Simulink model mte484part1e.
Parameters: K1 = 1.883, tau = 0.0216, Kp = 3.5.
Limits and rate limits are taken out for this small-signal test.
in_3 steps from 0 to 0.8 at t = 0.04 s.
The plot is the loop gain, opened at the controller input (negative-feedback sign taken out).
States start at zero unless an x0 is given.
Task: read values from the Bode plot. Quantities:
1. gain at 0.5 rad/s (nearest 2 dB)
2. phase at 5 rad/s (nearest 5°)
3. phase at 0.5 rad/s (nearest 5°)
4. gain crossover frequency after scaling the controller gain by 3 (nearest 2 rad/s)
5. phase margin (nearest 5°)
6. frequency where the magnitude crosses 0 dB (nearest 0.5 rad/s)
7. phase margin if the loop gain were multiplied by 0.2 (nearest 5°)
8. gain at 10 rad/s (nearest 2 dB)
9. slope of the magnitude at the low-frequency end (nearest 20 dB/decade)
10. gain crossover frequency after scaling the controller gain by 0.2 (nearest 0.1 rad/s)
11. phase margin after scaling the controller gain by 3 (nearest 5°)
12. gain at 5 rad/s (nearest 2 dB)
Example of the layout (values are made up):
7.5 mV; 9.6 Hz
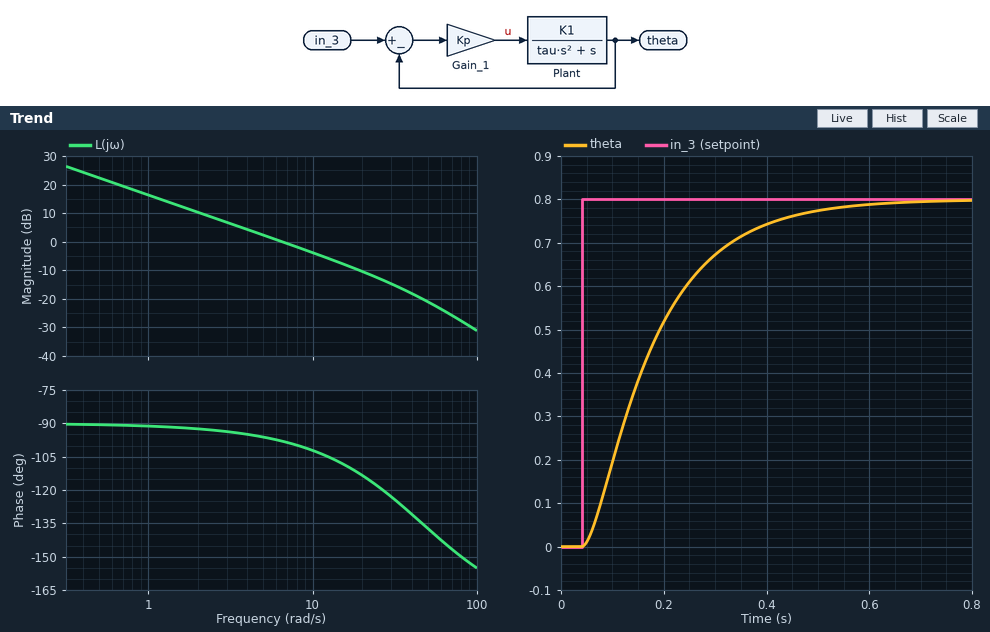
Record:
22 dB; -95°; -90°; 18 rad/s; 80°; 6.5 rad/s; 90°; -4 dB; -20 dB/decade; 1.3 rad/s; 70°; 2 dB
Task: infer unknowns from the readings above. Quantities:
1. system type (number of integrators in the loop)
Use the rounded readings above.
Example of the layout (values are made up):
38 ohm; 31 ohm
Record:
1
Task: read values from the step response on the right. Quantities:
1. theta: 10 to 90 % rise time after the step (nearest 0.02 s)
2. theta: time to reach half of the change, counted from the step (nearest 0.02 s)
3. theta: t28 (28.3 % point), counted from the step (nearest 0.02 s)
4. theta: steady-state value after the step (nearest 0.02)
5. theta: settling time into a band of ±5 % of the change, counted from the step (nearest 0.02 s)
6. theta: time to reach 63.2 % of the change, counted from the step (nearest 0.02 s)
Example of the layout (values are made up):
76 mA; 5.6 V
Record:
0.28 s; 0.12 s; 0.06 s; 0.80; 0.40 s; 0.16 s
